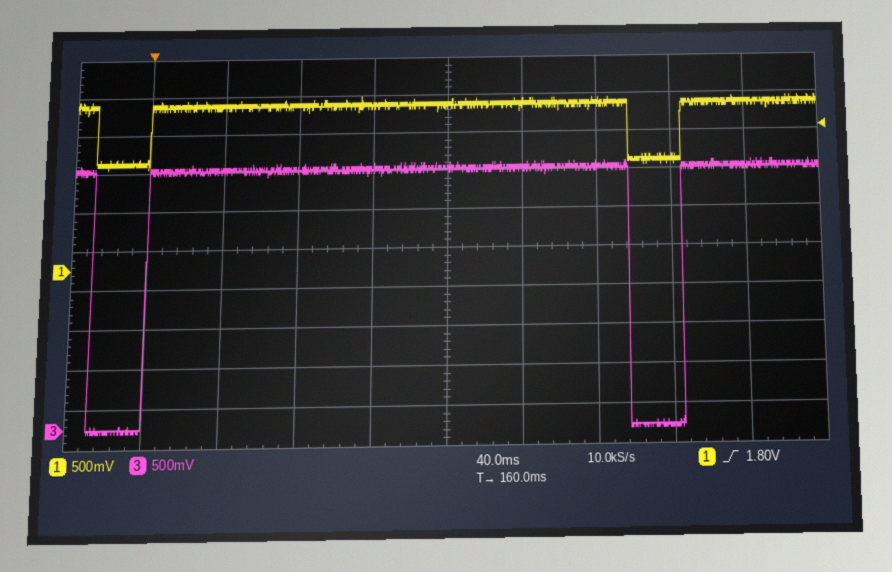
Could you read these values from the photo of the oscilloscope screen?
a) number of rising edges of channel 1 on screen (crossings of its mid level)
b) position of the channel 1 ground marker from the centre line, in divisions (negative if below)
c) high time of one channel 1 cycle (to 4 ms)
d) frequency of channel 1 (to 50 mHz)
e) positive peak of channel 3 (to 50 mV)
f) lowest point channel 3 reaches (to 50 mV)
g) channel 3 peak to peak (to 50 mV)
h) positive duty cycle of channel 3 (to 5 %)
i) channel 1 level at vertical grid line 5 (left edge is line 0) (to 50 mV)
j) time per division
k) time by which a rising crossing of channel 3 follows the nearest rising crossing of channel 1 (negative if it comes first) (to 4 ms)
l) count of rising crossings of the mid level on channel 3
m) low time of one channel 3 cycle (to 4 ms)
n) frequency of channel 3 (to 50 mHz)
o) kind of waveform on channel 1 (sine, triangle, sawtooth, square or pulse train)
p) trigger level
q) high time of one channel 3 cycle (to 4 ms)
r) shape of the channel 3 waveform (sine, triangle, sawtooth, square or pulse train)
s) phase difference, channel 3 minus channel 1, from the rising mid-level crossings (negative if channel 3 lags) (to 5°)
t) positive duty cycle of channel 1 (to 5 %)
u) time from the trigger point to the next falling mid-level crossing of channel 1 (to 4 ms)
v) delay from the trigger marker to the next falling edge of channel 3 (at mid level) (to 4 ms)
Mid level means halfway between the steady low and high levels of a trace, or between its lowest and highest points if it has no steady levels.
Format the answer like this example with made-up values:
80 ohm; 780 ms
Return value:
2; -0.5 div; 256 ms; 3.50 Hz; 3.35 V; -50 mV; 3.40 V; 90 %; 2.10 V; 40 ms; 0 ms; 2; 28 ms; 3.50 Hz; pulse train; 1.80 V; 256 ms; pulse train; 0°; 90 %; 256 ms; 256 ms
